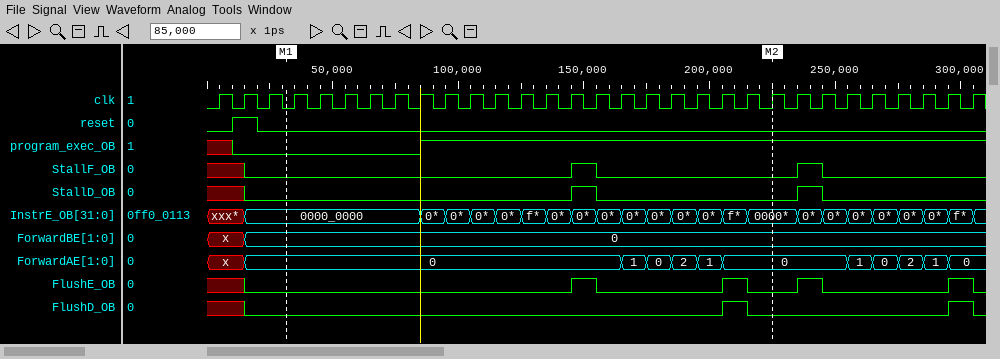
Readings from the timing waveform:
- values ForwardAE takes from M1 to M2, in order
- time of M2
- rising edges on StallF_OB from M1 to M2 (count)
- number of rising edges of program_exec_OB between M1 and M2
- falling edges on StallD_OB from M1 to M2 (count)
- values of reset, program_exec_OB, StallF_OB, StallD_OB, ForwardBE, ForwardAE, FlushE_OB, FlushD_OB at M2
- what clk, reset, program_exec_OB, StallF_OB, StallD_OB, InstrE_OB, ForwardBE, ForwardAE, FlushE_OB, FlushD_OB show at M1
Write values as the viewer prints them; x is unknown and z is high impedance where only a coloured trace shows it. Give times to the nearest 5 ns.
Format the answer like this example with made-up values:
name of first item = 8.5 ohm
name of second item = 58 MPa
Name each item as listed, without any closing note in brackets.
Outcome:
values ForwardAE takes from M1 to M2, in order = 0, 1, 0, 2, 1, 0
time of M2 = 225 ns
rising edges on StallF_OB from M1 to M2 = 1
number of rising edges of program_exec_OB between M1 and M2 = 1
falling edges on StallD_OB from M1 to M2 = 1
values of reset, program_exec_OB, StallF_OB, StallD_OB, ForwardBE, ForwardAE, FlushE_OB, FlushD_OB at M2 = reset=0, program_exec_OB=1, StallF_OB=0, StallD_OB=0, ForwardBE=0, ForwardAE=0, FlushE_OB=0, FlushD_OB=0
what clk, reset, program_exec_OB, StallF_OB, StallD_OB, InstrE_OB, ForwardBE, ForwardAE, FlushE_OB, FlushD_OB show at M1 = clk=0, reset=0, program_exec_OB=0, StallF_OB=0, StallD_OB=0, InstrE_OB=0000_0000, ForwardBE=0, ForwardAE=0, FlushE_OB=0, FlushD_OB=0
